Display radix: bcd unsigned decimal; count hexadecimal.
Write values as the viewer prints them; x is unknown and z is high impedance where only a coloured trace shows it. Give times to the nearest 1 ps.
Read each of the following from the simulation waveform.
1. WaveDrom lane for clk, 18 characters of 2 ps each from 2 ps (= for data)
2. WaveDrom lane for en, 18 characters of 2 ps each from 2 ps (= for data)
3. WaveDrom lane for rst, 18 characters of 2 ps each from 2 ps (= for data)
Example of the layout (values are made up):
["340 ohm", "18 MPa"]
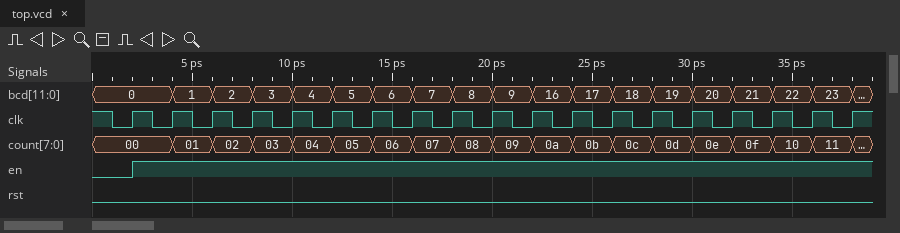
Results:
["{name: 'clk', wave: 'p.................'}", "{name: 'en', wave: '1.................'}", "{name: 'rst', wave: '0.................'}"]
